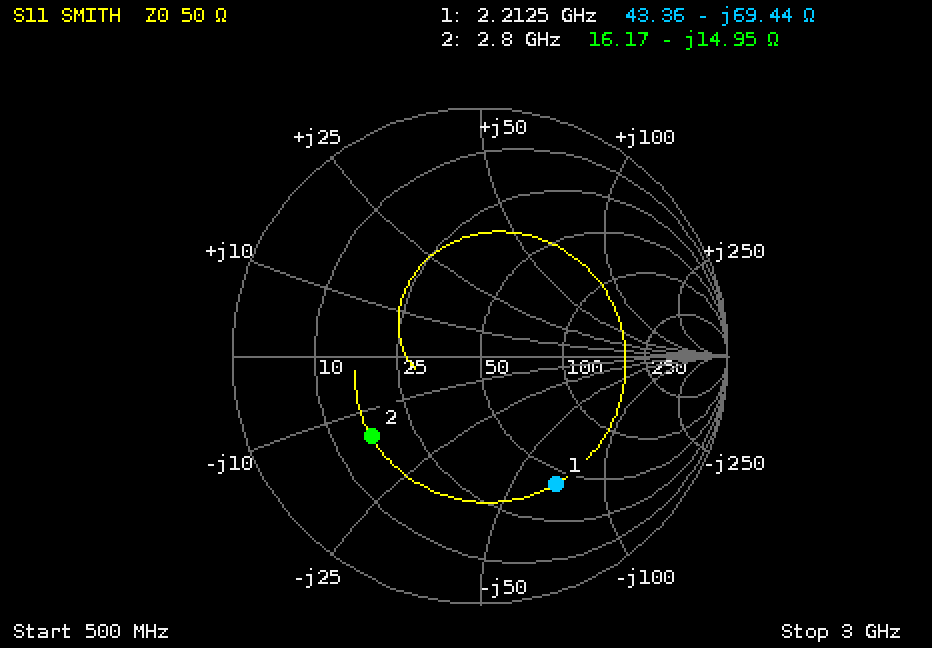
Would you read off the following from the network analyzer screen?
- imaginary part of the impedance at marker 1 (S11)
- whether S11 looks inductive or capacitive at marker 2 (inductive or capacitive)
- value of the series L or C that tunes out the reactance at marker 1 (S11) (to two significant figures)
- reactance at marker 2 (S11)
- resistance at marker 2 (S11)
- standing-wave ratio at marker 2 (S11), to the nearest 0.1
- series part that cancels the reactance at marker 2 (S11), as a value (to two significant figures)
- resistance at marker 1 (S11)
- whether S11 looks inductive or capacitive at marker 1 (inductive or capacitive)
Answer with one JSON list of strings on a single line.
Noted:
["-69.44 Ω", "capacitive", "5.0 nH", "-14.95 Ω", "16.17 Ω", "3.4", "850 pH", "43.36 Ω", "capacitive"]
